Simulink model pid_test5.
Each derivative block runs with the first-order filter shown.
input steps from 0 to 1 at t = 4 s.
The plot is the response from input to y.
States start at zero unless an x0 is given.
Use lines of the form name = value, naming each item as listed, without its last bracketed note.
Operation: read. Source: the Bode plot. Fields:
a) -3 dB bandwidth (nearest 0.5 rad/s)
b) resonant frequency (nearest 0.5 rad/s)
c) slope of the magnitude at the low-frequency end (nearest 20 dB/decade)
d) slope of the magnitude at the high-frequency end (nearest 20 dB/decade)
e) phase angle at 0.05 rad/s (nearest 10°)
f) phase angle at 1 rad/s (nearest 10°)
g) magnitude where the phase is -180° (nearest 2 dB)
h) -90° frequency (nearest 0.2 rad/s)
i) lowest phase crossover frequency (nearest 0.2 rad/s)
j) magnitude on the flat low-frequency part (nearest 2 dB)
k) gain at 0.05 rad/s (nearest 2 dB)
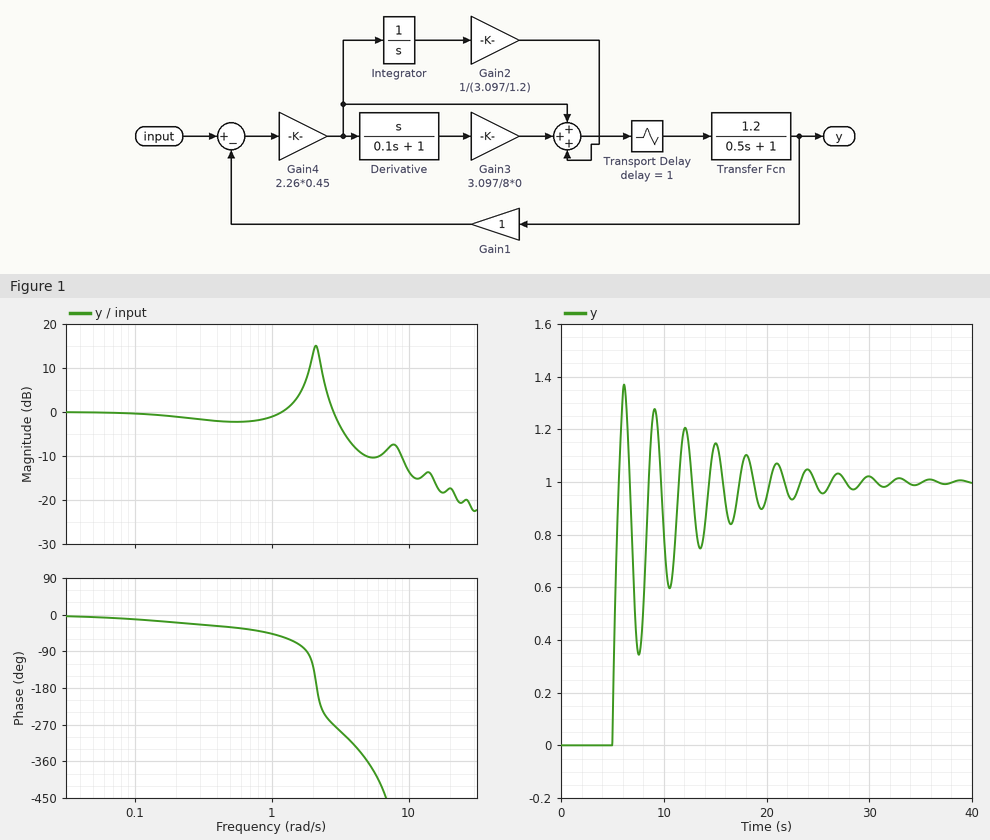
-3 dB bandwidth = 3.0 rad/s
resonant frequency = 2.0 rad/s
slope of the magnitude at the low-frequency end = 0 dB/decade
slope of the magnitude at the high-frequency end = -20 dB/decade
phase angle at 0.05 rad/s = -10°
phase angle at 1 rad/s = -50°
magnitude where the phase is -180° = 14 dB
-90° frequency = 1.8 rad/s
lowest phase crossover frequency = 2.2 rad/s
magnitude on the flat low-frequency part = 0 dB
gain at 0.05 rad/s = 0 dB
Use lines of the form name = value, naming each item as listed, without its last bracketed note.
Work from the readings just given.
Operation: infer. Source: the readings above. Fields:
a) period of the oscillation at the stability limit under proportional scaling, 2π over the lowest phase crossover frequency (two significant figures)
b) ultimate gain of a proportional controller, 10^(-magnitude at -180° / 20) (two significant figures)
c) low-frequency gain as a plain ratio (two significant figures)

period of the oscillation at the stability limit under proportional scaling, 2π over the lowest phase crossover frequency = 2.9 s
ultimate gain of a proportional controller, 10^(-magnitude at -180° / 20) = 0.20
low-frequency gain as a plain ratio = 1.0
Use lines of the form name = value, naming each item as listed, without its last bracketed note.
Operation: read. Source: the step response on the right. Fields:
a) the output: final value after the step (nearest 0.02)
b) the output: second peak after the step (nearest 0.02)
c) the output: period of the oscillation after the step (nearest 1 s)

the output: final value after the step = 1.00
the output: second peak after the step = 1.28
the output: period of the oscillation after the step = 3 s
